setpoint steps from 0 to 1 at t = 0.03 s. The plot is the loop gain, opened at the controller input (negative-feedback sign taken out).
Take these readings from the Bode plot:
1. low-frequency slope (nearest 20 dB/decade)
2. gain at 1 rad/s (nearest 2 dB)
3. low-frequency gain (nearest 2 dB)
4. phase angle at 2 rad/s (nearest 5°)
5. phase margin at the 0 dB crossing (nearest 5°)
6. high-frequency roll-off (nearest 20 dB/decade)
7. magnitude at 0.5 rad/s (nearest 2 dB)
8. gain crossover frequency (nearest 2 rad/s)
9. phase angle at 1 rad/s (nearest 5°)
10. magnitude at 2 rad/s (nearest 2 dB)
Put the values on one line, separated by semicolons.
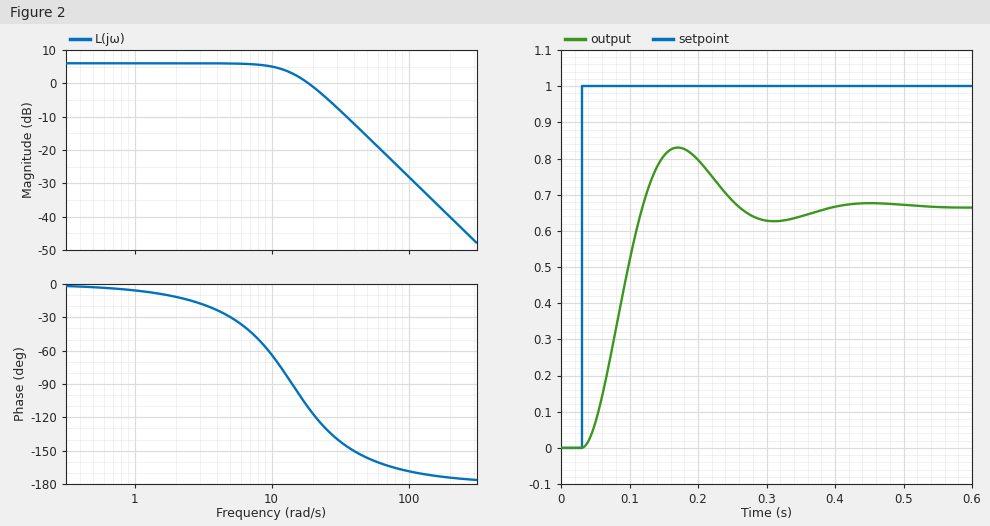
0 dB/decade; 6 dB; 6 dB; -10°; 70°; -40 dB/decade; 6 dB; 18 rad/s; -5°; 6 dB
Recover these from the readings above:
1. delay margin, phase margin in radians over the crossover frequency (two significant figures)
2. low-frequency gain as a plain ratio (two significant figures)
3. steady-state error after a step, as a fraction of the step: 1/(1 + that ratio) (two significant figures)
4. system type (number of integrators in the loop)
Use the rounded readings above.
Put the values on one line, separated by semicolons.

0.068 s; 2.0; 0.33; 0
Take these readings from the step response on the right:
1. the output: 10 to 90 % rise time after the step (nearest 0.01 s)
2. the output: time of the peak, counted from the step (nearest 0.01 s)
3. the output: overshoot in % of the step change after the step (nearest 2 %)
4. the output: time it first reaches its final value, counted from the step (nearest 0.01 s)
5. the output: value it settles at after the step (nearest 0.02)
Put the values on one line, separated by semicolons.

0.06 s; 0.14 s; 24 %; 0.09 s; 0.66
